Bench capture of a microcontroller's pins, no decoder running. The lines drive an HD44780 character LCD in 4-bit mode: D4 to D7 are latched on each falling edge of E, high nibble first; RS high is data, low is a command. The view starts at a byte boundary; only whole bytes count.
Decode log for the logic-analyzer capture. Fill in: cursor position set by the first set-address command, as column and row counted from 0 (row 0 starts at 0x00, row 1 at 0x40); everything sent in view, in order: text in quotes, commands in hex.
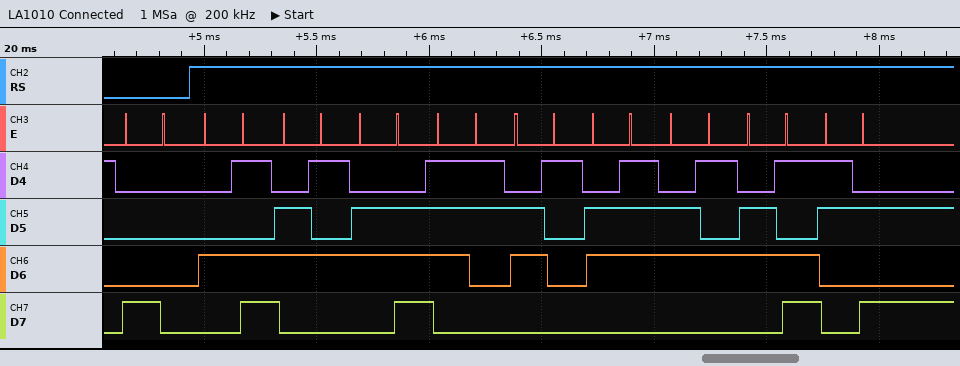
column 0, row 0
0x80 "Mensagem:"
